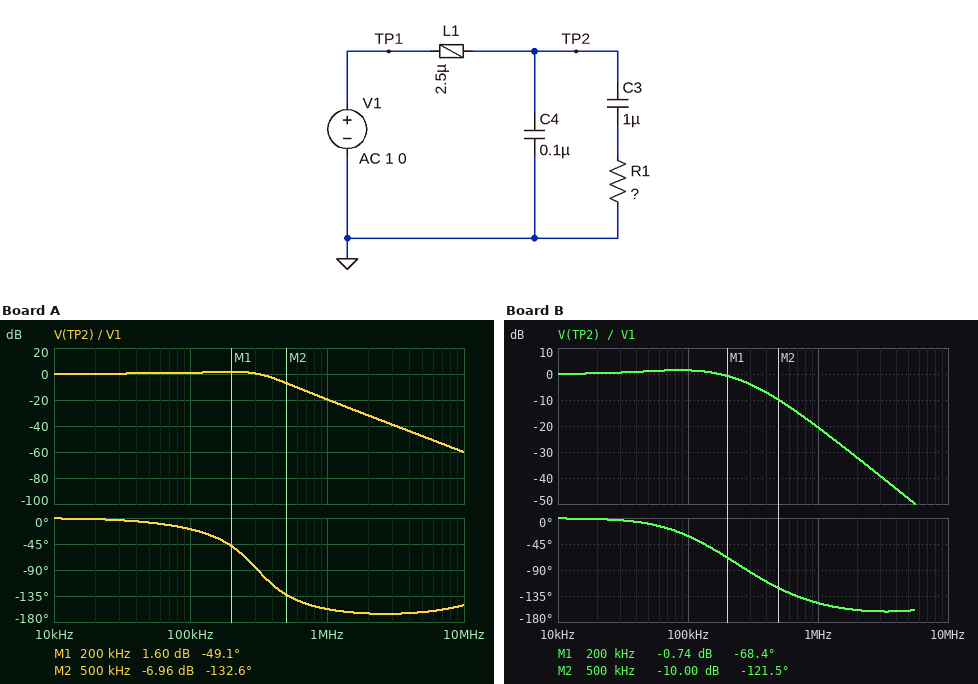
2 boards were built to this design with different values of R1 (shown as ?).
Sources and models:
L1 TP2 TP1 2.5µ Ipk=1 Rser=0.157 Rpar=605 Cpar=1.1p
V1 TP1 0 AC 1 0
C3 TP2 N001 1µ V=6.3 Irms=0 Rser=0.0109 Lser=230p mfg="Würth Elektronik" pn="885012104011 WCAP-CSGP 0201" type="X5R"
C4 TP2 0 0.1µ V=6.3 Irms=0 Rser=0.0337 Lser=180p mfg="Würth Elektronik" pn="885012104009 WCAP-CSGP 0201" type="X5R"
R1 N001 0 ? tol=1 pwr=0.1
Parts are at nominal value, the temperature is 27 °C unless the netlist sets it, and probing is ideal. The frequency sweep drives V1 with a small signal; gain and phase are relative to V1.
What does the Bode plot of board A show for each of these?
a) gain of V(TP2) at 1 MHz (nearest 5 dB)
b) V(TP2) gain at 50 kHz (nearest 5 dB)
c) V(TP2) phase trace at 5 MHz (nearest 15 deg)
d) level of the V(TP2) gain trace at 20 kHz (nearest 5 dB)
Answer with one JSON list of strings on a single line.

["-20 dB", "0 dB", "-165 deg", "0 dB"]
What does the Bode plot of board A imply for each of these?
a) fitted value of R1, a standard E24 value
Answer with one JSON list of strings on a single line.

["5.1 Ω"]
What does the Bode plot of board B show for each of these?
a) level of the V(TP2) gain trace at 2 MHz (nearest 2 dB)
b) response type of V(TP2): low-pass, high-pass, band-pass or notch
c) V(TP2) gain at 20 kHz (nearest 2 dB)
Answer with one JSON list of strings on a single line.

["-32 dB", "low-pass", "0 dB"]
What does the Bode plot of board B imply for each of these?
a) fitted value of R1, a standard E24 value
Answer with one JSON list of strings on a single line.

["3 Ω"]
